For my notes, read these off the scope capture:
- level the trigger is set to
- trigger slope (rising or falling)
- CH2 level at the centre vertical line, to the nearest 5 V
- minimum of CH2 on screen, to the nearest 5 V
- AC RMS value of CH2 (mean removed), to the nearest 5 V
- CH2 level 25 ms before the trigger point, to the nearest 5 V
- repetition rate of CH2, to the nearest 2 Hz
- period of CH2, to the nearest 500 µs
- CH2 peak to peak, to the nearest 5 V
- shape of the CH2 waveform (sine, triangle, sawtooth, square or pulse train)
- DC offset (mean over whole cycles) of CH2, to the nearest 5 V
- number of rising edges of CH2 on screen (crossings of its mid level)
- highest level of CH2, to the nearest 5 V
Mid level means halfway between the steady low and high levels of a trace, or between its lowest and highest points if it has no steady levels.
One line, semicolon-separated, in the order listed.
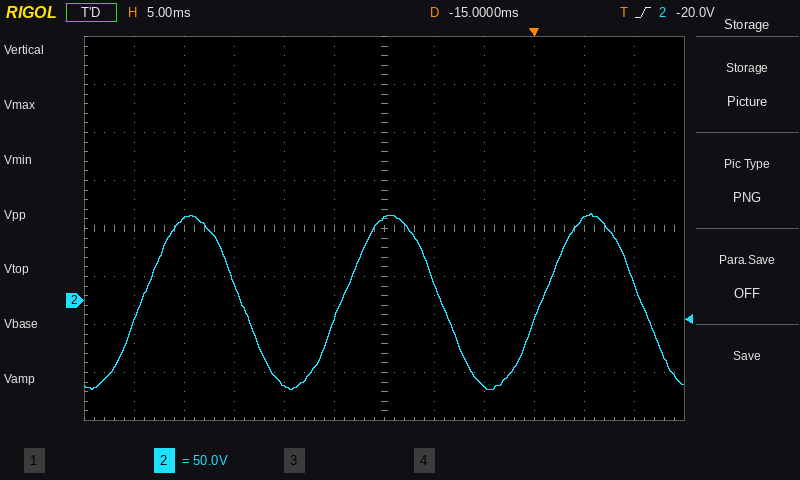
-20.0 V; rising; 85 V; -95 V; 65 V; -90 V; 50 Hz; 20.0 ms; 185 V; sine; 0 V; 3; 90 V
